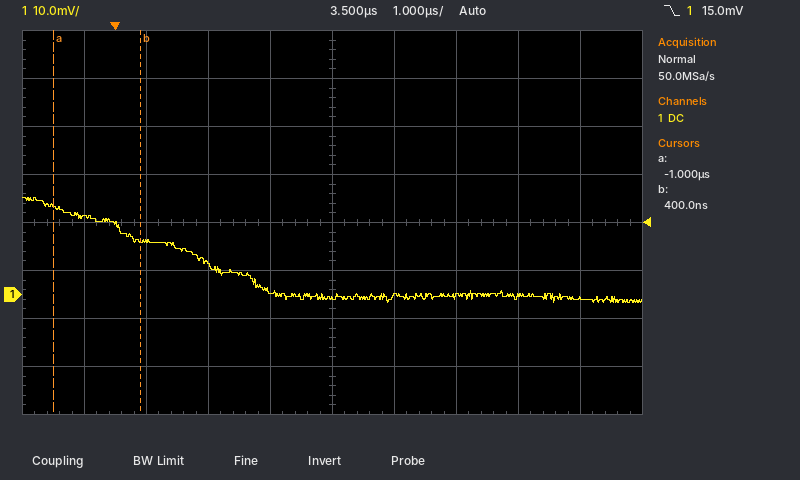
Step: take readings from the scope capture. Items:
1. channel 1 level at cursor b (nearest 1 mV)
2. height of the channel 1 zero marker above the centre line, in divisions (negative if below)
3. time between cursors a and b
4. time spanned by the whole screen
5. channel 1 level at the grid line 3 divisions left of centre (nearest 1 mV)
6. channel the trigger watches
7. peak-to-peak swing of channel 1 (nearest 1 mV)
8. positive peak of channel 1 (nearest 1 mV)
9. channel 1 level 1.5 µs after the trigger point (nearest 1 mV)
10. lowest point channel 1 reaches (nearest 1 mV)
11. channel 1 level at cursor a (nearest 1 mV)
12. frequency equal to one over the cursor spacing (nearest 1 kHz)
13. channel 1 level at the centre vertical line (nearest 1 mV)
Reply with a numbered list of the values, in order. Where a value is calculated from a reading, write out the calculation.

1. 11 mV
2. -1.5 div
3. 400 ns − (-1 µs) = 1.4 µs
4. 10 µs
5. 11 mV
6. channel 1
7. 20 mV − (-2 mV) = 22 mV
8. 20 mV
9. 6 mV
10. -2 mV
11. 18 mV
12. 1 / 1.4 µs ≈ 714 kHz
13. -1 mV
